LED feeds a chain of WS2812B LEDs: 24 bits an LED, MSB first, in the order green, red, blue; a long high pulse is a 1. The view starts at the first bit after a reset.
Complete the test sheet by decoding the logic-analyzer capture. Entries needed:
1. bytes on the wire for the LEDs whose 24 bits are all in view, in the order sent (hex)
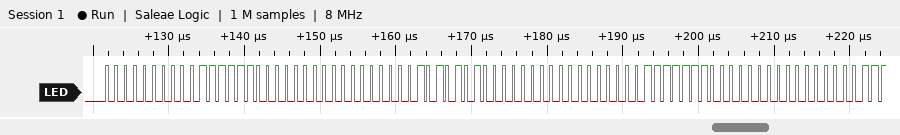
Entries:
00 3F 00 00 55 00 00 7F 00
